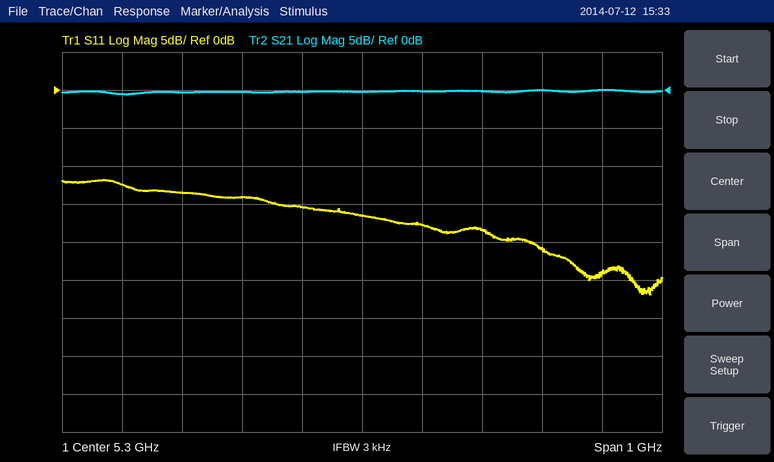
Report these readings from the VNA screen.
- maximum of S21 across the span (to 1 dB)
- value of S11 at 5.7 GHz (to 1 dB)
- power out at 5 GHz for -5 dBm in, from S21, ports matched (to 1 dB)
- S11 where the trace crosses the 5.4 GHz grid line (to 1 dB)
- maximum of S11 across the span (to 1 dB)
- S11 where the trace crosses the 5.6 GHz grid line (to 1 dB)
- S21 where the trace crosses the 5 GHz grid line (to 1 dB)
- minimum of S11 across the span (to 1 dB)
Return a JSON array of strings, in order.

["0 dB", "-24 dB", "-5 dBm", "-18 dB", "-12 dB", "-21 dB", "0 dB", "-27 dB"]
